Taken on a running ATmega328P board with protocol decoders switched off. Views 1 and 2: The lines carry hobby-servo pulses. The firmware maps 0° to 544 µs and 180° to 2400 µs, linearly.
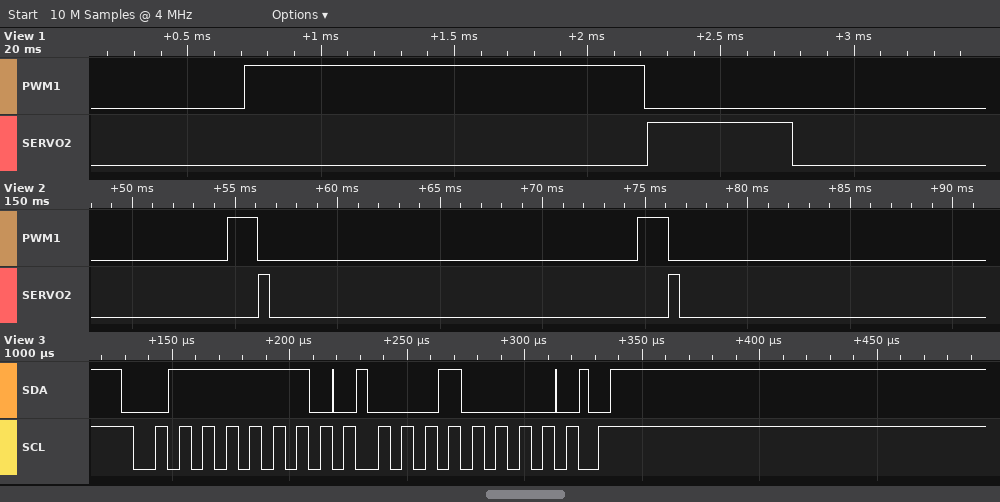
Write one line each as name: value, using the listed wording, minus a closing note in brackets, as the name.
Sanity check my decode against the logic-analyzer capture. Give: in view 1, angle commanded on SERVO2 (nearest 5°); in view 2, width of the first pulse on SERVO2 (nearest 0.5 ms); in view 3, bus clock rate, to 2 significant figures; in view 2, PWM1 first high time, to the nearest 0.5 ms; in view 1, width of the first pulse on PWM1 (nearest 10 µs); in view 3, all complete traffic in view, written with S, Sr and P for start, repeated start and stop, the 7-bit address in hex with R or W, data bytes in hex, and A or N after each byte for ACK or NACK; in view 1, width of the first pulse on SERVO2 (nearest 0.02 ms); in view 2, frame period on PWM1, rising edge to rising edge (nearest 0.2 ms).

in view 1, angle commanded on SERVO2: 0°
in view 2, width of the first pulse on SERVO2: 0.5 ms
in view 3, bus clock rate, to 2 significant figures: 100 kHz
in view 2, PWM1 first high time, to the nearest 0.5 ms: 1.5 ms
in view 1, width of the first pulse on PWM1: 1500 µs
in view 3, all complete traffic in view, written with S, Sr and P for start, repeated start and stop, the 7-bit address in hex with R or W, data bytes in hex, and A or N after each byte for ACK or NACK: S 3FW A 10 A P
in view 1, width of the first pulse on SERVO2: 0.54 ms
in view 2, frame period on PWM1, rising edge to rising edge: 20.0 ms
